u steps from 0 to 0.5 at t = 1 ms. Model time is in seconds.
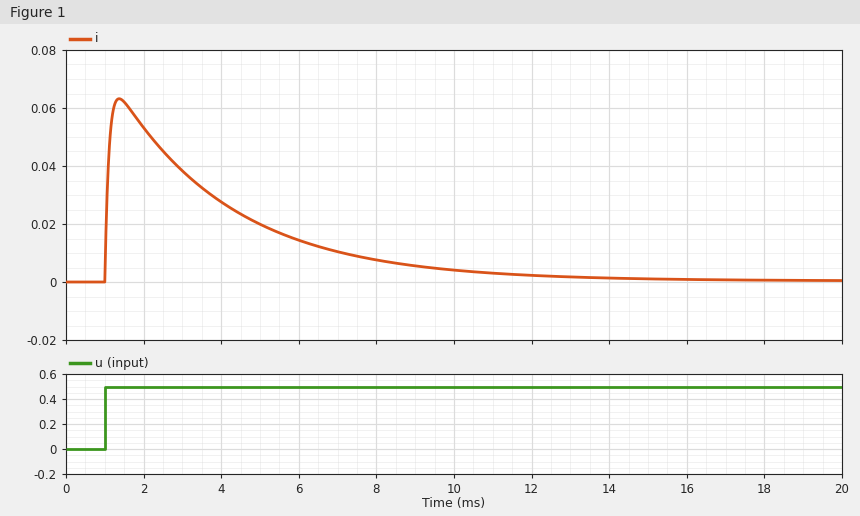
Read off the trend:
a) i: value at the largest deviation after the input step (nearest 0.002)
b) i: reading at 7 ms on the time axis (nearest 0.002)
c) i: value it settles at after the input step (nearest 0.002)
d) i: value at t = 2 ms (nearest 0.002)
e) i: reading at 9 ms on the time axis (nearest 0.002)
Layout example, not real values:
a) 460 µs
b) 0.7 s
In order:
a) 0.064
b) 0.010
c) 0.000
d) 0.054
e) 0.006
